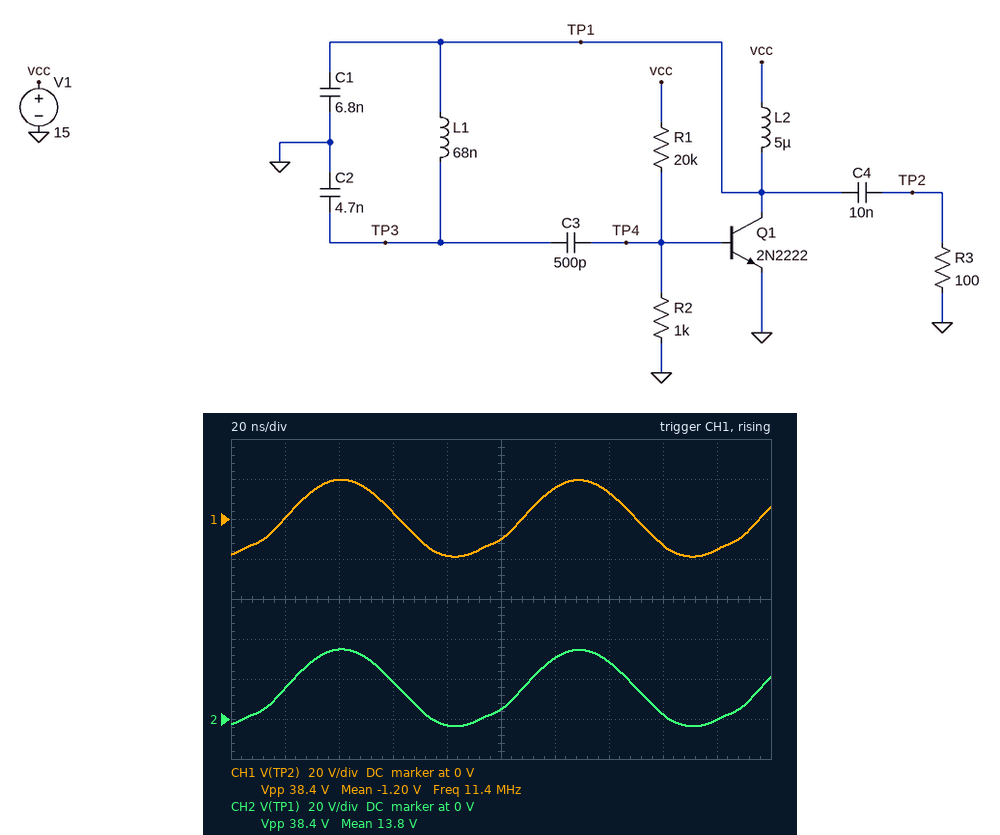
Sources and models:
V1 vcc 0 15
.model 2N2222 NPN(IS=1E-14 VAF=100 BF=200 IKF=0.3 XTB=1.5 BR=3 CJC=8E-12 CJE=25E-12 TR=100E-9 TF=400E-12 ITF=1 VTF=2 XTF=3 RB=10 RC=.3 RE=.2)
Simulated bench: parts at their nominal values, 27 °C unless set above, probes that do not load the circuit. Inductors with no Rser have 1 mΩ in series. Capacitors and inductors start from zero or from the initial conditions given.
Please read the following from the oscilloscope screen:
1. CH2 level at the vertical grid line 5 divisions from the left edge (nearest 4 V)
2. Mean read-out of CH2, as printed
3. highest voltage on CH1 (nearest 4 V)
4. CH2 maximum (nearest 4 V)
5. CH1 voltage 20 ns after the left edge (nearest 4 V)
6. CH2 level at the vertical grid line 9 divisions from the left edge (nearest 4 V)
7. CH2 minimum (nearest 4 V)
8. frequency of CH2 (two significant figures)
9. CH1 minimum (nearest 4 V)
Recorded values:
4 V
13.8 V
20 V
36 V
0 V
0 V
-4 V
11 MHz
-20 V
